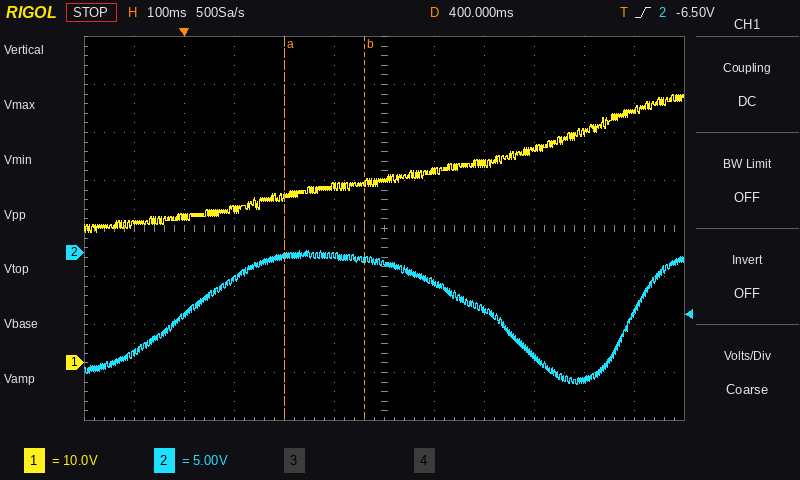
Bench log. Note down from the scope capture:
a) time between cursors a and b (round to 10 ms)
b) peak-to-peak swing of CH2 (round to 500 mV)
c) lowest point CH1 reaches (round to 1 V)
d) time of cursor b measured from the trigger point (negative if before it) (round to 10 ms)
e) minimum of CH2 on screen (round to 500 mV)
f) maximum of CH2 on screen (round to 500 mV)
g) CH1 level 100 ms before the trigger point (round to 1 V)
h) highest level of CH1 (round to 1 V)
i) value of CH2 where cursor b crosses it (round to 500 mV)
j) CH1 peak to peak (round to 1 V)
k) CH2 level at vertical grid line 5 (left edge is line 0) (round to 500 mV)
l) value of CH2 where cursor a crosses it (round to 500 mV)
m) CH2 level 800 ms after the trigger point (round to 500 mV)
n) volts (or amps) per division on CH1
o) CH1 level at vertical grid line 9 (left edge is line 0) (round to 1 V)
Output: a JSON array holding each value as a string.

["160 ms", "14.0 V", "27 V", "+360 ms", "-14.0 V", "0.0 V", "29 V", "56 V", "-500 mV", "29 V", "-500 mV", "-500 mV", "-13.0 V", "10 V", "45 V"]
